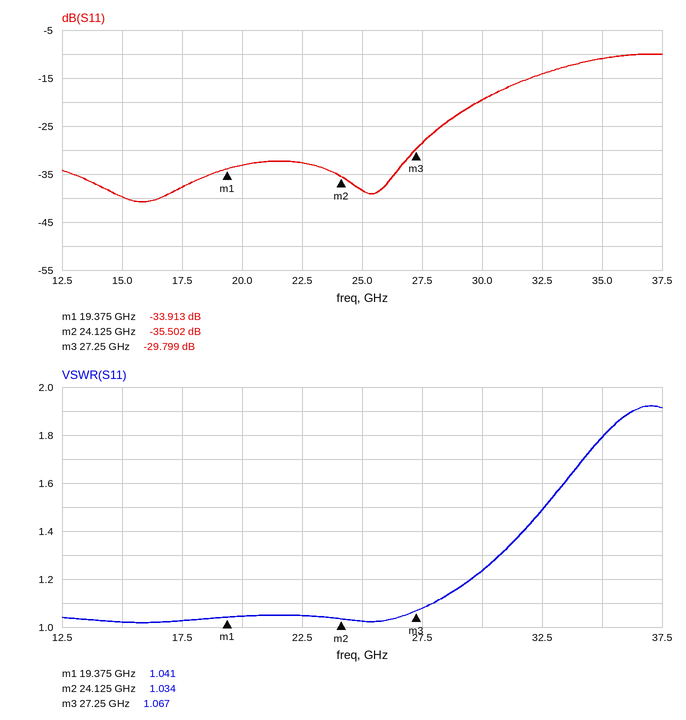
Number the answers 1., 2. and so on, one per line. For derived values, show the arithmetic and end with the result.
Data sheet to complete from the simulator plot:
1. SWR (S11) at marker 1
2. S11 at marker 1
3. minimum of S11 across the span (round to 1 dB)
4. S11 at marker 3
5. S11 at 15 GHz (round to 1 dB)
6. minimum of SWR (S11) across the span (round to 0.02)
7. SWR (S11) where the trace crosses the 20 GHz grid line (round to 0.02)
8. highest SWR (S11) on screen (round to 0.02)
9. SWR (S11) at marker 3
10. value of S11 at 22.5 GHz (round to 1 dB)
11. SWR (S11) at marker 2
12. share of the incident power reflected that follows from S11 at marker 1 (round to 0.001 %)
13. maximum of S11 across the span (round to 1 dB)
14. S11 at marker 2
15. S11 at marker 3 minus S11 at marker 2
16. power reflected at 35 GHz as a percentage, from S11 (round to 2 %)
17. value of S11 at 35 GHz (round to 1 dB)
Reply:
1. 1.041
2. -33.913 dB
3. -41 dB
4. -29.799 dB
5. -40 dB
6. 1.02
7. 1.04
8. 1.92
9. 1.067
10. -33 dB
11. 1.034
12. 10^(-33.913/10) ≈ 0.041 %
13. -10 dB
14. -35.502 dB
15. -29.799 − (-35.502) = 5.703 dB
16. 10^(-11/10) ≈ 8 %
17. -11 dB
